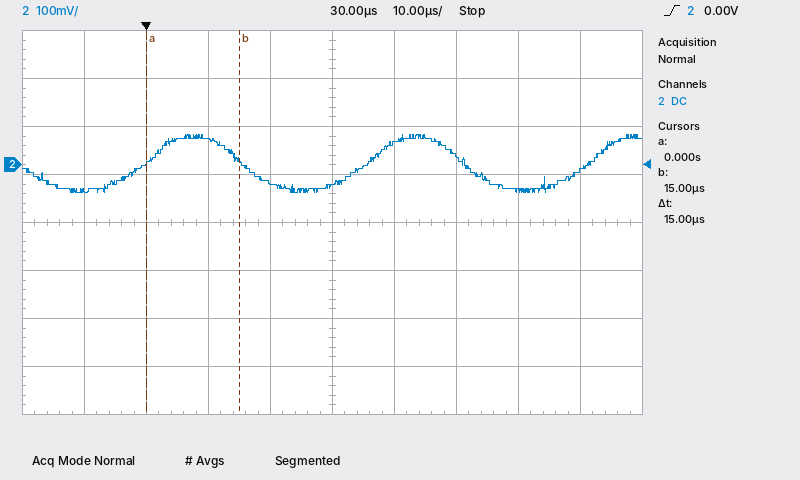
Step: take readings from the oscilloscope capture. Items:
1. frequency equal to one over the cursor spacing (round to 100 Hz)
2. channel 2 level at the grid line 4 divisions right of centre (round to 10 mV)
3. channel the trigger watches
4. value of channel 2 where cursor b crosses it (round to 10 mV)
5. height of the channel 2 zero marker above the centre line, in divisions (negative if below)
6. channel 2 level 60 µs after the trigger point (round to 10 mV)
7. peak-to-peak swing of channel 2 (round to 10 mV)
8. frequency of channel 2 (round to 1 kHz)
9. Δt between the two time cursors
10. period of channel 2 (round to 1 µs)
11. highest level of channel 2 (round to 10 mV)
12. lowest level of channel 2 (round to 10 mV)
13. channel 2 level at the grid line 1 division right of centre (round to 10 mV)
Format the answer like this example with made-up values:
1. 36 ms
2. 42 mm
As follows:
1. 66.7 kHz
2. -10 mV
3. channel 2
4. 10 mV
5. +1.2 div
6. -50 mV
7. 120 mV
8. 28 kHz
9. 15 µs
10. 36 µs
11. 60 mV
12. -60 mV
13. 40 mV
